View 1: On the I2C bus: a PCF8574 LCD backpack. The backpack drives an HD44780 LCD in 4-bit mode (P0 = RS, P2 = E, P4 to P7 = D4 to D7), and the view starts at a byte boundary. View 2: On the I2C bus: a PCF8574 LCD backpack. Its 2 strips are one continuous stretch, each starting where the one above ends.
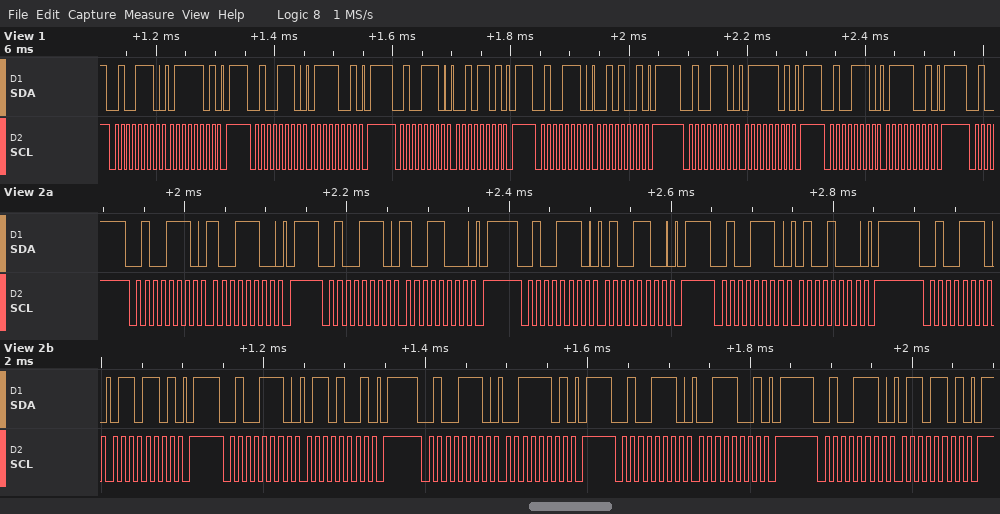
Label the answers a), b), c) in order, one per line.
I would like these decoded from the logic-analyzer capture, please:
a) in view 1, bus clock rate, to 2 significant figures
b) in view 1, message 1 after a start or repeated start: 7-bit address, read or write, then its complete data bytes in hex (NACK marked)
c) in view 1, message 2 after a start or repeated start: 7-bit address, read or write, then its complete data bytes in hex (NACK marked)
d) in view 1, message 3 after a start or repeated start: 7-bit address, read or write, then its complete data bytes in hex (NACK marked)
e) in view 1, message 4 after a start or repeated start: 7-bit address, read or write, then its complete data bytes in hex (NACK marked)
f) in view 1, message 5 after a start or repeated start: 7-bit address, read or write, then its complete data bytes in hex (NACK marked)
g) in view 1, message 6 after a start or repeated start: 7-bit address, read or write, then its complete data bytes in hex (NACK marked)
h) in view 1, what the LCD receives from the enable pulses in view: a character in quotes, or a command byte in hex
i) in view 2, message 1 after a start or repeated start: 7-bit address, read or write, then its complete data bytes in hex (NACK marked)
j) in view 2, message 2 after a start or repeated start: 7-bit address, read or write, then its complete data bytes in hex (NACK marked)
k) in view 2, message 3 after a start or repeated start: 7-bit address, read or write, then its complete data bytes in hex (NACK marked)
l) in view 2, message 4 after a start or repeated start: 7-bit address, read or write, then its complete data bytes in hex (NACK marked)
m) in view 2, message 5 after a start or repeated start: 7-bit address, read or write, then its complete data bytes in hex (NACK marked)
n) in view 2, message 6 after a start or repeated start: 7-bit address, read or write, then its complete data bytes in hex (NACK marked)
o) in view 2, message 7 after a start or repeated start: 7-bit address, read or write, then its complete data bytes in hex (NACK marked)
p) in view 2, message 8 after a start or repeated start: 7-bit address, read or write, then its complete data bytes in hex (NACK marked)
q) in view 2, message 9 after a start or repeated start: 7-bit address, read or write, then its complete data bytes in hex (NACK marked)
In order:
a) 100 kHz
b) 0x27 write: 7D
c) 0x27 write: 79
d) 0x27 write: 2D
e) 0x27 write: 29
f) 0x27 write: 7D
g) 0x27 write: 79
h) 'r'
i) 0x27 write: 9C
j) 0x27 write: 98
k) 0x27 write: 4C
l) 0x27 write: 48
m) 0x27 write: 6D
n) 0x27 write: 69
o) 0x27 write: 3D
p) 0x27 write: 39
q) 0x27 write: 6D
